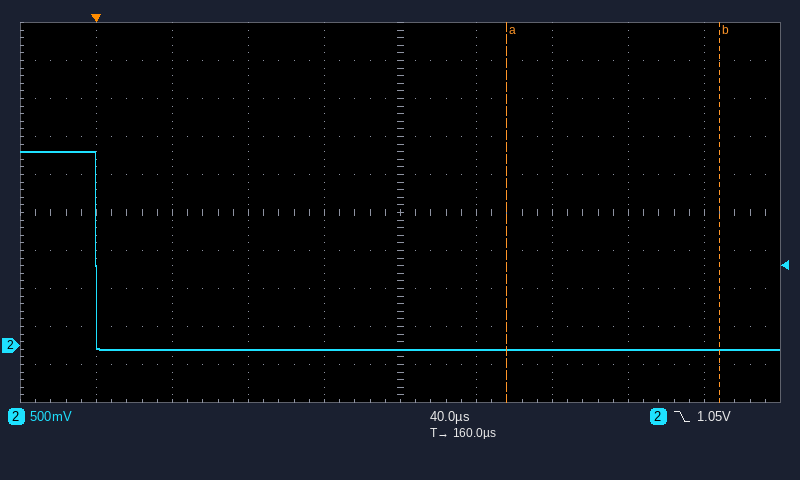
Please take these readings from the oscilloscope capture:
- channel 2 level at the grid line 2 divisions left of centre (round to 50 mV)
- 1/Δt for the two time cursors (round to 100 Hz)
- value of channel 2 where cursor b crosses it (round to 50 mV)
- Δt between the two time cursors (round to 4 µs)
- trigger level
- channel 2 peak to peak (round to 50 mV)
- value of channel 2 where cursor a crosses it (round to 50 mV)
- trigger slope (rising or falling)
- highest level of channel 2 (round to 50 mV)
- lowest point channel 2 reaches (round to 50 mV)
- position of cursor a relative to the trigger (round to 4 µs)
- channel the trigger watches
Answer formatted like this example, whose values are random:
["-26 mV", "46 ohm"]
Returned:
["-50 mV", "8.9 kHz", "-50 mV", "112 µs", "1.05 V", "2.60 V", "-50 mV", "falling", "2.55 V", "-50 mV", "+216 µs", "channel 2"]
